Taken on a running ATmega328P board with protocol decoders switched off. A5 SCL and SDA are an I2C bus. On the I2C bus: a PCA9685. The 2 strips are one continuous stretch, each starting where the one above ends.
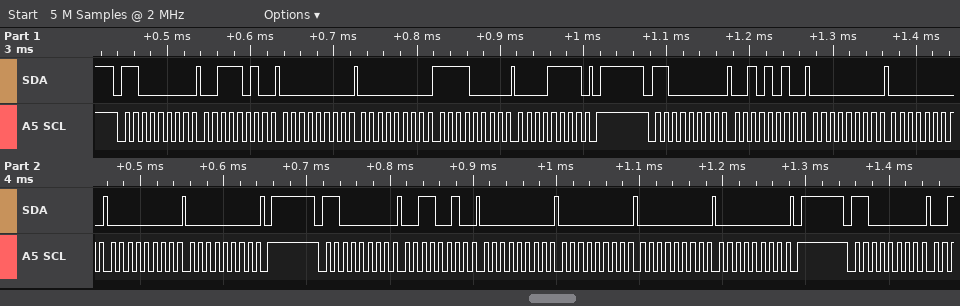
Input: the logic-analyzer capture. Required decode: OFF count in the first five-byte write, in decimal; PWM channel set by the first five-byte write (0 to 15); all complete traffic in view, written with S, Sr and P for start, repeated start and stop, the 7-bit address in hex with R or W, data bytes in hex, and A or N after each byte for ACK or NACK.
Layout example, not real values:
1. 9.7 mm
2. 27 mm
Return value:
1. 4080
2. 13
3. S 60W A 3A A 00 A 00 A F0 A 0F A P S 60W A 2A A 00 A 00 A 00 A 00 A P S 60W A 32 A 00 A 00 A 00 A 00 A P S 60W A
